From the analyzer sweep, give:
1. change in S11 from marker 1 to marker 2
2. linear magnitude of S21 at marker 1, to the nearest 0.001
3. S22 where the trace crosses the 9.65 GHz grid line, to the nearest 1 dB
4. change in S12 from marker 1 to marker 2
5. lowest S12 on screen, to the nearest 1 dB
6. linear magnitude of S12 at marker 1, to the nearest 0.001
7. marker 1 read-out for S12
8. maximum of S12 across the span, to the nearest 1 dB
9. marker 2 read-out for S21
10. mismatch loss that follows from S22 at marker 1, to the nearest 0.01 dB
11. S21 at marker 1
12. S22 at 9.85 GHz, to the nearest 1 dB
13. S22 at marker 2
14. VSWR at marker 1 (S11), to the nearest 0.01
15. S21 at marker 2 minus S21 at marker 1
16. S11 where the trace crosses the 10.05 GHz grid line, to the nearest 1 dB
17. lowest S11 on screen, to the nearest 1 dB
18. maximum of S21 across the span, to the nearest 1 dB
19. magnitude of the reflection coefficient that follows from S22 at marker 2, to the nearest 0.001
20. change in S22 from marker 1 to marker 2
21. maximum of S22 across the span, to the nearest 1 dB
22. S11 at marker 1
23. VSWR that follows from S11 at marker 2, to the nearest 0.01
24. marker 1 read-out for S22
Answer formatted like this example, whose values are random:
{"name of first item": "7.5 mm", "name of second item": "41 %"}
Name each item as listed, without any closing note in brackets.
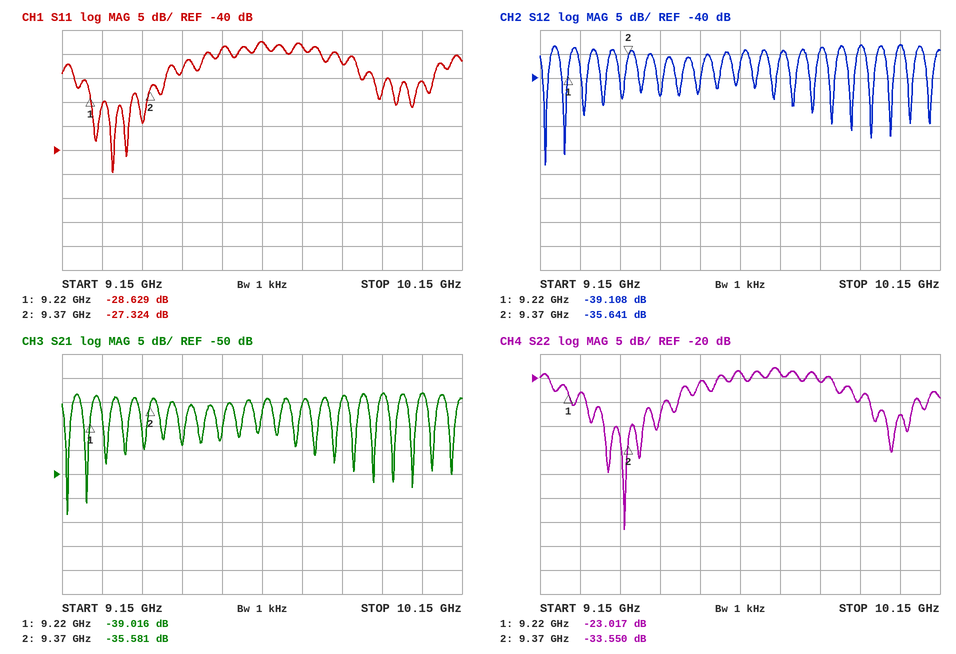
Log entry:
{"change in S11 from marker 1 to marker 2": "1.305 dB", "linear magnitude of S21 at marker 1, to the nearest 0.001": "0.011", "S22 where the trace crosses the 9.65 GHz grid line, to the nearest 1 dB": "-19 dB", "change in S12 from marker 1 to marker 2": "3.467 dB", "lowest S12 on screen, to the nearest 1 dB": "-58 dB", "linear magnitude of S12 at marker 1, to the nearest 0.001": "0.011", "marker 1 read-out for S12": "-39.108 dB", "maximum of S12 across the span, to the nearest 1 dB": "-33 dB", "marker 2 read-out for S21": "-35.581 dB", "mismatch loss that follows from S22 at marker 1, to the nearest 0.01 dB": "0.02 dB", "S21 at marker 1": "-39.016 dB", "S22 at 9.85 GHz, to the nearest 1 dB": "-21 dB", "S22 at marker 2": "-33.550 dB", "VSWR at marker 1 (S11), to the nearest 0.01": "1.08", "S21 at marker 2 minus S21 at marker 1": "3.435 dB", "S11 where the trace crosses the 10.05 GHz grid line, to the nearest 1 dB": "-26 dB", "lowest S11 on screen, to the nearest 1 dB": "-45 dB", "maximum of S21 across the span, to the nearest 1 dB": "-33 dB", "magnitude of the reflection coefficient that follows from S22 at marker 2, to the nearest 0.001": "0.021", "change in S22 from marker 1 to marker 2": "-10.533 dB", "maximum of S22 across the span, to the nearest 1 dB": "-18 dB", "S11 at marker 1": "-28.629 dB", "VSWR that follows from S11 at marker 2, to the nearest 0.01": "1.09", "marker 1 read-out for S22": "-23.017 dB"}
